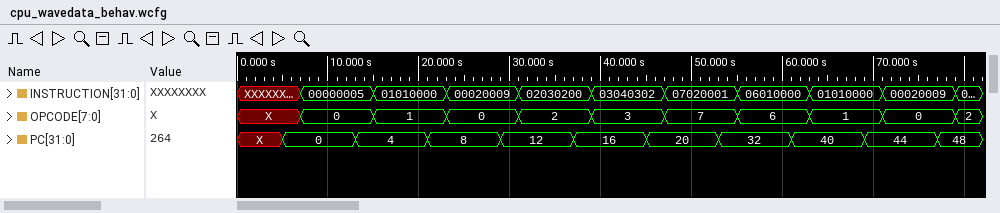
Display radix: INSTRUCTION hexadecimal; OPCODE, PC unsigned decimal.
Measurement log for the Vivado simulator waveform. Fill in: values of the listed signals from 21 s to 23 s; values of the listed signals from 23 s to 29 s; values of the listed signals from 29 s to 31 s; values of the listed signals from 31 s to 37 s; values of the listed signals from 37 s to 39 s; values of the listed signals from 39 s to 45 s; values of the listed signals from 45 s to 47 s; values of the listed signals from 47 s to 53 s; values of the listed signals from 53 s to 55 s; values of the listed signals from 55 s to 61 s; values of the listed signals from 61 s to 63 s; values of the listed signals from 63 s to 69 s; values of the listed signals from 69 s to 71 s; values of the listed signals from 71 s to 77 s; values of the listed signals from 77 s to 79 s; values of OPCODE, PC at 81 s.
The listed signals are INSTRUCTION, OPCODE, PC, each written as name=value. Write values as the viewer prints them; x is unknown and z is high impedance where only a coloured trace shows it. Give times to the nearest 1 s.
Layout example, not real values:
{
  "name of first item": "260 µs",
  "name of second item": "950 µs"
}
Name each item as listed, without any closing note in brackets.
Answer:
{
  "values of the listed signals from 21 s to 23 s": "INSTRUCTION=01010000, OPCODE=1, PC=8",
  "values of the listed signals from 23 s to 29 s": "INSTRUCTION=00020009, OPCODE=0, PC=8",
  "values of the listed signals from 29 s to 31 s": "INSTRUCTION=00020009, OPCODE=0, PC=12",
  "values of the listed signals from 31 s to 37 s": "INSTRUCTION=02030200, OPCODE=2, PC=12",
  "values of the listed signals from 37 s to 39 s": "INSTRUCTION=02030200, OPCODE=2, PC=16",
  "values of the listed signals from 39 s to 45 s": "INSTRUCTION=03040302, OPCODE=3, PC=16",
  "values of the listed signals from 45 s to 47 s": "INSTRUCTION=03040302, OPCODE=3, PC=20",
  "values of the listed signals from 47 s to 53 s": "INSTRUCTION=07020001, OPCODE=7, PC=20",
  "values of the listed signals from 53 s to 55 s": "INSTRUCTION=07020001, OPCODE=7, PC=32",
  "values of the listed signals from 55 s to 61 s": "INSTRUCTION=06010000, OPCODE=6, PC=32",
  "values of the listed signals from 61 s to 63 s": "INSTRUCTION=06010000, OPCODE=6, PC=40",
  "values of the listed signals from 63 s to 69 s": "INSTRUCTION=01010000, OPCODE=1, PC=40",
  "values of the listed signals from 69 s to 71 s": "INSTRUCTION=01010000, OPCODE=1, PC=44",
  "values of the listed signals from 71 s to 77 s": "INSTRUCTION=00020009, OPCODE=0, PC=44",
  "values of the listed signals from 77 s to 79 s": "INSTRUCTION=00020009, OPCODE=0, PC=48",
  "values of OPCODE, PC at 81 s": "OPCODE=2, PC=48"
}
